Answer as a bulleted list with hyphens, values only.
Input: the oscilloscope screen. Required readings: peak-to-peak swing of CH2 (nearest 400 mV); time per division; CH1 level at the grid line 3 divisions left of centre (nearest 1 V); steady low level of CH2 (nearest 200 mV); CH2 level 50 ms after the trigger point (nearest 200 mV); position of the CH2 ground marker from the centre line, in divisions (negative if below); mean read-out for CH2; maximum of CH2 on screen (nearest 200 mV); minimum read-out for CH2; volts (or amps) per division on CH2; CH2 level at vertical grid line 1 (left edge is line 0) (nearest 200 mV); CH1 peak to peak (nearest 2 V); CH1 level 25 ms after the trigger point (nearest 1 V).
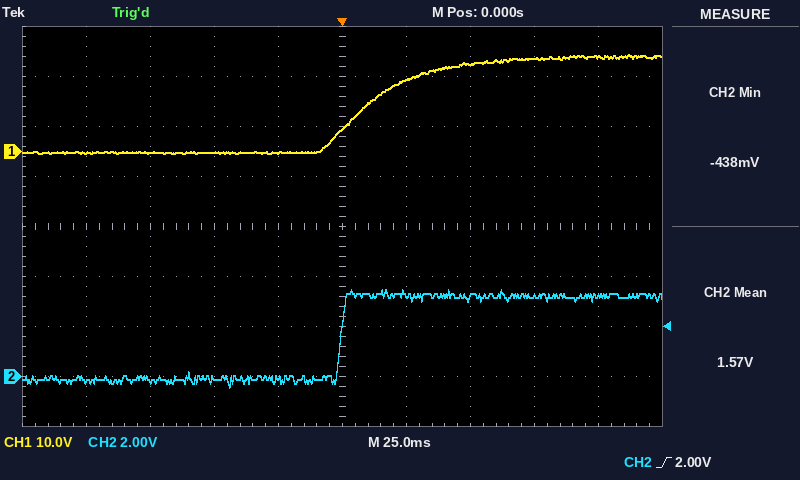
- 4.0 V
- 25 ms
- 0 V
- -200 mV
- 3.2 V
- -3.0 div
- 1.57 V
- 3.4 V
- -438 mV
- 2 V
- -200 mV
- 20 V
- 14 V
